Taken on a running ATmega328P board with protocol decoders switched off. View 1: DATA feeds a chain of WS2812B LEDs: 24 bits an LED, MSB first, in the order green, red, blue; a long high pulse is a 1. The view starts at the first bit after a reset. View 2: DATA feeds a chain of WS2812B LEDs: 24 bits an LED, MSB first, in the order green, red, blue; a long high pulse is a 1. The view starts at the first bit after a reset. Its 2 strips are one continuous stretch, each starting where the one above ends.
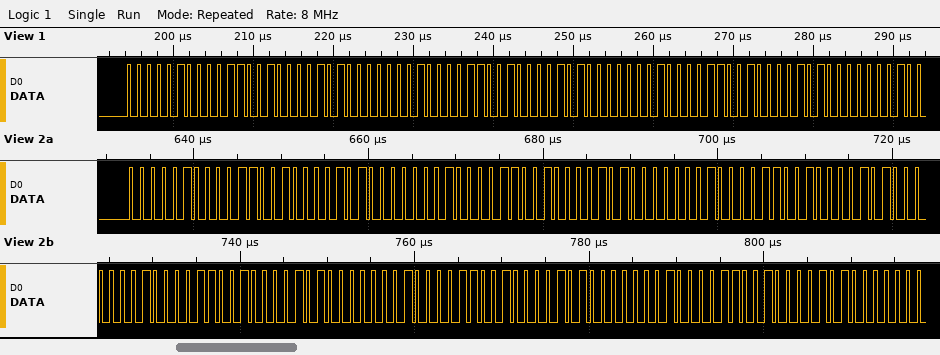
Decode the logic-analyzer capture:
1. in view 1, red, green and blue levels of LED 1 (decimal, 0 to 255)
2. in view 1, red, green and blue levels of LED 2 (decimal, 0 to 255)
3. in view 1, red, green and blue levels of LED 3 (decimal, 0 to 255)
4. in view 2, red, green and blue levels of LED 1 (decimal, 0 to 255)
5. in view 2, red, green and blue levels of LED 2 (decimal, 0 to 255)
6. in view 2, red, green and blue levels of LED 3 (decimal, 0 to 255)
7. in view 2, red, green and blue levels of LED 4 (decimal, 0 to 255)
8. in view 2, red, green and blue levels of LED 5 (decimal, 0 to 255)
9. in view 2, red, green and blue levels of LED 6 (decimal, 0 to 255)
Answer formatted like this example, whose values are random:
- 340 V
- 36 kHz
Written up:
- 50, 4, 20
- 50, 4, 20
- 50, 4, 20
- 50, 4, 20
- 50, 4, 20
- 50, 4, 20
- 50, 4, 20
- 50, 4, 20
- 50, 4, 20
